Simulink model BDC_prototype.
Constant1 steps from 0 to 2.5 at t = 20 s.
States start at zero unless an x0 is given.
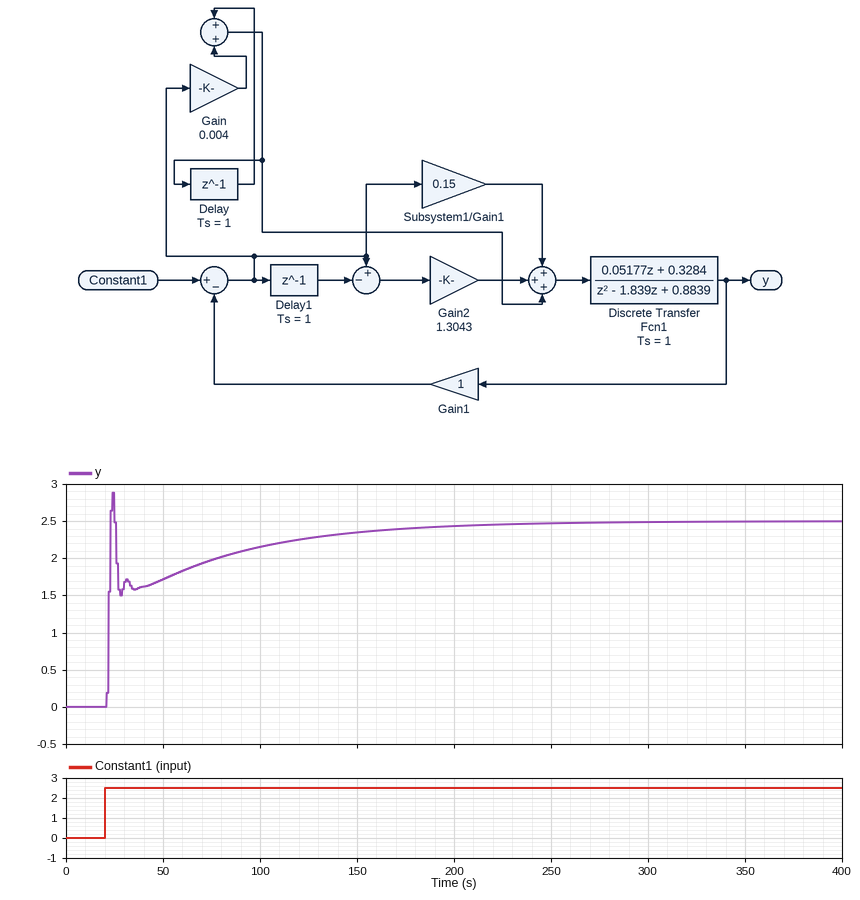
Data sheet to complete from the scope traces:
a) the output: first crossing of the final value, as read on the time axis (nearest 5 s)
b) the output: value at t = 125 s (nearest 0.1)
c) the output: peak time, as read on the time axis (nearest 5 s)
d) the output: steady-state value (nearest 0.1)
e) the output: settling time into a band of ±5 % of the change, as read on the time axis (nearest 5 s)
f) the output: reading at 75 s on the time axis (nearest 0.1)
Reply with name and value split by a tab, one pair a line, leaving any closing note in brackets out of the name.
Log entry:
the output: first crossing of the final value, as read on the time axis	25 s
the output: value at t = 125 s	2.3
the output: peak time, as read on the time axis	25 s
the output: steady-state value	2.5
the output: settling time into a band of ±5 % of the change, as read on the time axis	160 s
the output: reading at 75 s on the time axis	2.0
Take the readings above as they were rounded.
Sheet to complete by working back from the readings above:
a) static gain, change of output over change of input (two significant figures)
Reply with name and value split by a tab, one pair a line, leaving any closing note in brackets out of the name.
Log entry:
static gain, change of output over change of input	1.0
